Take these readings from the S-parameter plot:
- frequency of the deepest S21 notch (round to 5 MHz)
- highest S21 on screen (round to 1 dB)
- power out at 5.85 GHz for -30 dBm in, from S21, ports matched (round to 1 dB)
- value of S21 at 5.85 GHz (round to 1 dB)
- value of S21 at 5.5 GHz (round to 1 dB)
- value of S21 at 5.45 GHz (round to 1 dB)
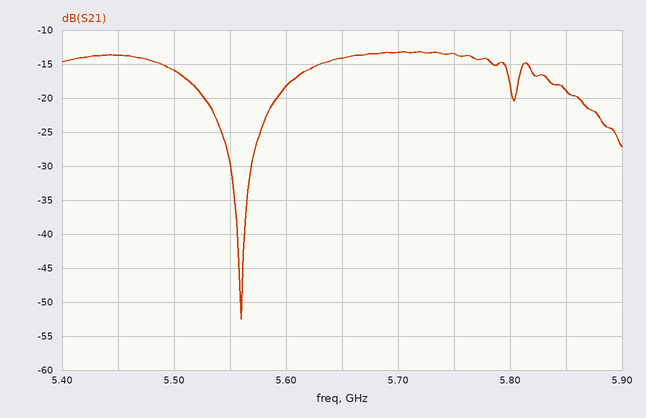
5.560 GHz
-13 dB
-49 dBm
-19 dB
-16 dB
-14 dB
